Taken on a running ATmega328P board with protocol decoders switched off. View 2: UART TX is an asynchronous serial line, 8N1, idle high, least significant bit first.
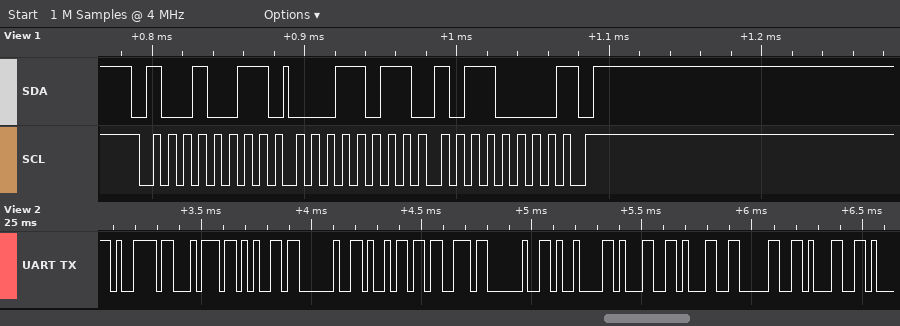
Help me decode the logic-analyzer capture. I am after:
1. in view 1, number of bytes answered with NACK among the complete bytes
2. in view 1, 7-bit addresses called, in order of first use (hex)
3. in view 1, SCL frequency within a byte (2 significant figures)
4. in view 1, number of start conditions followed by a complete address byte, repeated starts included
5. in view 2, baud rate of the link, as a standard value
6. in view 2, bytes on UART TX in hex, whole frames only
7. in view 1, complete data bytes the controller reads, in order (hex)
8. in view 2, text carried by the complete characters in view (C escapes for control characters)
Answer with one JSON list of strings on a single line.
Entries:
["1", "0x49", "100 kHz", "1", "38400 baud", "0x79 0x74 0x65 0x20 0x69 0x73 0x20 0x09 0x31 0x31 0x30 0x31", "1B B0", "\"yte is \\t1101\""]
